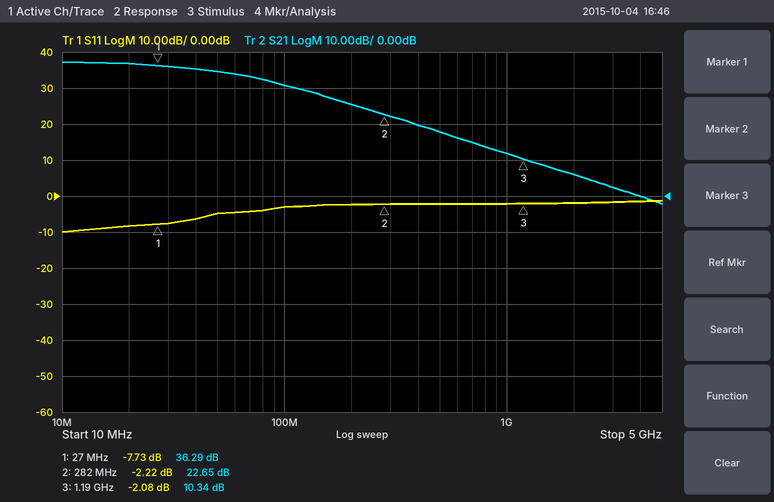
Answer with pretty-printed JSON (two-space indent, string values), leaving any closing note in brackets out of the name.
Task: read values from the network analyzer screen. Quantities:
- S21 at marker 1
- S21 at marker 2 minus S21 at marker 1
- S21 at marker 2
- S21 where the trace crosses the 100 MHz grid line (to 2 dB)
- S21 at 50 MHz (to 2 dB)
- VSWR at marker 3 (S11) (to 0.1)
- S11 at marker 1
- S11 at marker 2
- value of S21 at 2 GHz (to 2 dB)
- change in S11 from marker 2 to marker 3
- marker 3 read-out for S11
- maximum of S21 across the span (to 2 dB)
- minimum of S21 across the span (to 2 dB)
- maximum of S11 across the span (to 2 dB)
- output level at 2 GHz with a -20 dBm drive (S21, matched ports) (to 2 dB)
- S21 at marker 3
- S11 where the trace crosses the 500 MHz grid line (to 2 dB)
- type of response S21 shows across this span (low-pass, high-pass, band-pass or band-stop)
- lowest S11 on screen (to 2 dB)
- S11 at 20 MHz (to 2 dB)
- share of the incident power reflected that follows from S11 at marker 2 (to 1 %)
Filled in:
{
  "S21 at marker 1": "36.29 dB",
  "S21 at marker 2 minus S21 at marker 1": "-13.64 dB",
  "S21 at marker 2": "22.65 dB",
  "S21 where the trace crosses the 100 MHz grid line": "30 dB",
  "S21 at 50 MHz": "34 dB",
  "VSWR at marker 3 (S11)": "8.4",
  "S11 at marker 1": "-7.73 dB",
  "S11 at marker 2": "-2.22 dB",
  "value of S21 at 2 GHz": "6 dB",
  "change in S11 from marker 2 to marker 3": "0.14 dB",
  "marker 3 read-out for S11": "-2.08 dB",
  "maximum of S21 across the span": "38 dB",
  "minimum of S21 across the span": "-2 dB",
  "maximum of S11 across the span": "-2 dB",
  "output level at 2 GHz with a -20 dBm drive (S21, matched ports)": "-14 dBm",
  "S21 at marker 3": "10.34 dB",
  "S11 where the trace crosses the 500 MHz grid line": "-2 dB",
  "type of response S21 shows across this span": "low-pass",
  "lowest S11 on screen": "-10 dB",
  "S11 at 20 MHz": "-8 dB",
  "share of the incident power reflected that follows from S11 at marker 2": "60 %"
}
